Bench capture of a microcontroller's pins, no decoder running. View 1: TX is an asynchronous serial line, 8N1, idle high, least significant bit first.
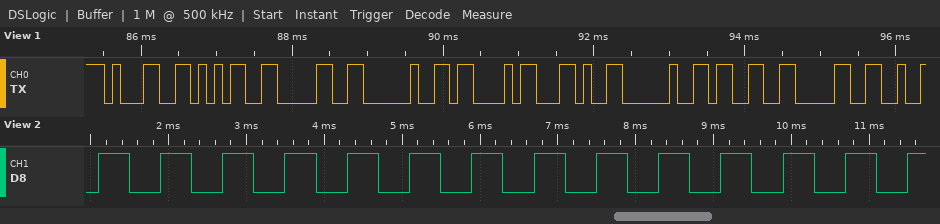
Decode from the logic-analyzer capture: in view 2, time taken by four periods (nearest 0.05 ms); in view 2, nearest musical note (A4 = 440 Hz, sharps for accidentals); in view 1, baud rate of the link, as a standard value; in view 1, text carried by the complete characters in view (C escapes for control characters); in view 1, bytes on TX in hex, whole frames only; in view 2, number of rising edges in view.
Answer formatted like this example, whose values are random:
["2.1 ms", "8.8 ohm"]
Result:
["3.20 ms", "D#6", "9600 baud", "\"150 C, 30\"", "0x31 0x35 0x30 0x20 0x43 0x2C 0x20 0x33 0x30", "14"]
